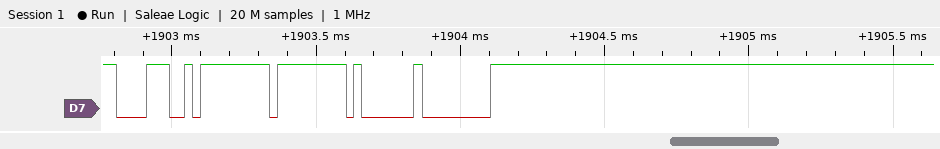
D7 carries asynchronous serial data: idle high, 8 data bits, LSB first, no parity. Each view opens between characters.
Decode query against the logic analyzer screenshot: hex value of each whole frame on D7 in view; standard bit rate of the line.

38, FF, FF, 01, 00
38400 baud
